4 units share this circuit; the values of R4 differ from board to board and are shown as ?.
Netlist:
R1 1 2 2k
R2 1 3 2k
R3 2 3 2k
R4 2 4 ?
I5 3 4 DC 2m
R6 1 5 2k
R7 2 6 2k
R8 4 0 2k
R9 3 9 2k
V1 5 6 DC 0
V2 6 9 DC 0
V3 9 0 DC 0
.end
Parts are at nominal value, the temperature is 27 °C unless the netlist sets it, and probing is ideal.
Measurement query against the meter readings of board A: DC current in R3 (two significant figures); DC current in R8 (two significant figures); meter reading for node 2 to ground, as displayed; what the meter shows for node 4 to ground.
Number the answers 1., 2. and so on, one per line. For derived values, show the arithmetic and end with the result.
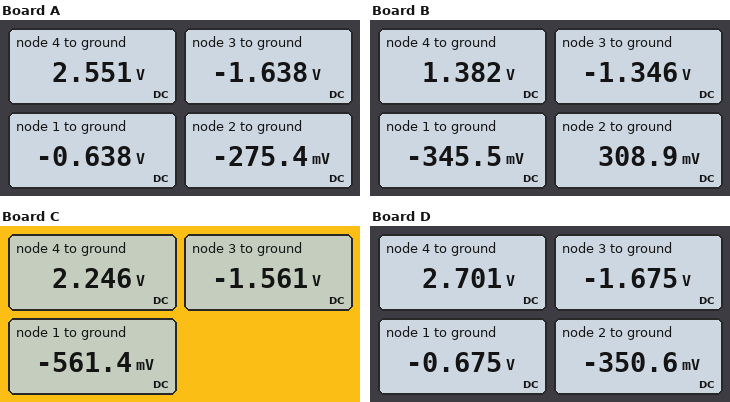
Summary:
1. (-275.4 mV - (-1.638 V)) / 2 kΩ = 680 µA
2. (2.551 V) / 2 kΩ = 1.3 mA
3. -275.4 mV
4. 2.551 V
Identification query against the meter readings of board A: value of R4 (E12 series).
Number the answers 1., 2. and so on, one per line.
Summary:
1. 3.9 kΩ
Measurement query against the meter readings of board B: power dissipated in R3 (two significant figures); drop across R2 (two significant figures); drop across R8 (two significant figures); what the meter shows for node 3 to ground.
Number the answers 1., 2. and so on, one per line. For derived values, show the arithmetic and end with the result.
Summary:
1. (308.9 mV - (-1.346 V))^2 / 2 kΩ = 1.4 mW
2. -345.5 mV - (-1.346 V) = 1.0 V
3. 1.382 V = 1.4 V
4. -1.346 V
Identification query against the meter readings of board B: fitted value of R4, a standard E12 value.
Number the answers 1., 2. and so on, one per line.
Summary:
1. 820 Ω
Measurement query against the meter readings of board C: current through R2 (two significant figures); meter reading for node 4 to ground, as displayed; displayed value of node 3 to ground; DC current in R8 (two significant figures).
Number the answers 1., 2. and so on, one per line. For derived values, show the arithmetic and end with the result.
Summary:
1. (-561.4 mV - (-1.561 V)) / 2 kΩ = 500 µA
2. 2.246 V
3. -1.561 V
4. (2.246 V) / 2 kΩ = 1.1 mA
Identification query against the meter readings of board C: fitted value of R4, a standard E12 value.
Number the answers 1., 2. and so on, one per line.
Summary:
1. 2.7 kΩ
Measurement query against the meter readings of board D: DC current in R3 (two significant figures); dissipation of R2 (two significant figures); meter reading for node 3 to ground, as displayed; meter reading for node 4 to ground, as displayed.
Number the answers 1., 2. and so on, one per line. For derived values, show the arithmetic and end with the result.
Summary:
1. (-350.6 mV - (-1.675 V)) / 2 kΩ = 660 µA
2. (-675 mV - (-1.675 V))^2 / 2 kΩ = 500 µW
3. -1.675 V
4. 2.701 V
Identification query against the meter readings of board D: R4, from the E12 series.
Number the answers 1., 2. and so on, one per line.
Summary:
1. 4.7 kΩ
